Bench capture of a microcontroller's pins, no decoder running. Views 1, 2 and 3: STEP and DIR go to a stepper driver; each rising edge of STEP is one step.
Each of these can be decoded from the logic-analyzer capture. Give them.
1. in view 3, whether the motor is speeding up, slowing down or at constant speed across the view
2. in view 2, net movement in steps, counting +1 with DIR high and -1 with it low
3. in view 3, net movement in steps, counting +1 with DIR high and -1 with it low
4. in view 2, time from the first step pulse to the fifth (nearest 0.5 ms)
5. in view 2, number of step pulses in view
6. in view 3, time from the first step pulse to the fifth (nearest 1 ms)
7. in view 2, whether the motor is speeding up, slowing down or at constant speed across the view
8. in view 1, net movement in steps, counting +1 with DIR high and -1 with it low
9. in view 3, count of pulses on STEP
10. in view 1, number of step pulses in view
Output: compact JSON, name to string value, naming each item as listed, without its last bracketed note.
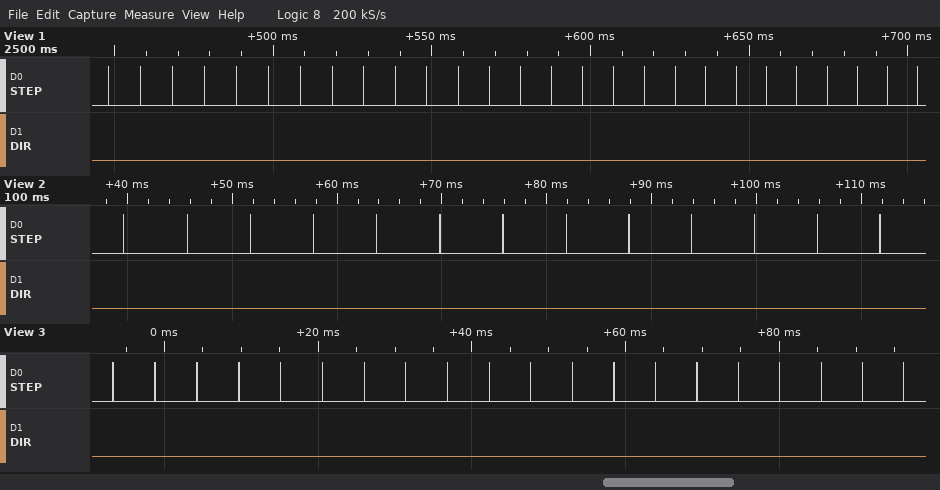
{"in view 3, whether the motor is speeding up, slowing down or at constant speed across the view": "constant speed", "in view 2, net movement in steps, counting +1 with DIR high and -1 with it low": "-13", "in view 3, net movement in steps, counting +1 with DIR high and -1 with it low": "-20", "in view 2, time from the first step pulse to the fifth": "24.0 ms", "in view 2, number of step pulses in view": "13", "in view 3, time from the first step pulse to the fifth": "22 ms", "in view 2, whether the motor is speeding up, slowing down or at constant speed across the view": "constant speed", "in view 1, net movement in steps, counting +1 with DIR high and -1 with it low": "-27", "in view 3, count of pulses on STEP": "20", "in view 1, number of step pulses in view": "27"}
